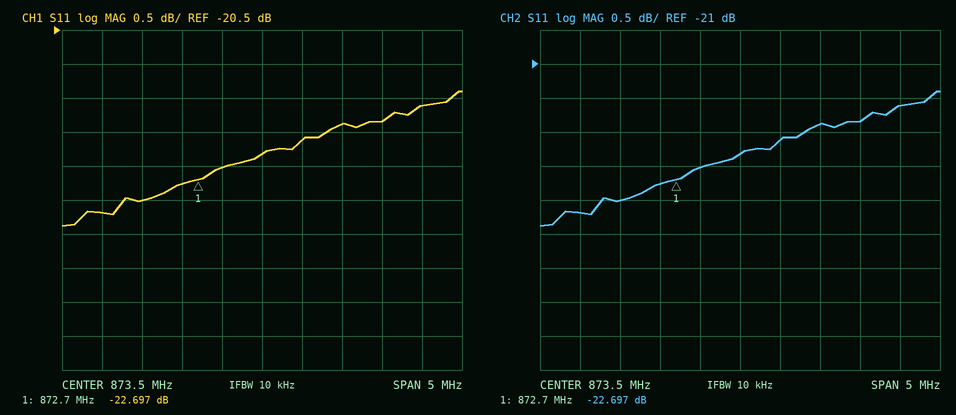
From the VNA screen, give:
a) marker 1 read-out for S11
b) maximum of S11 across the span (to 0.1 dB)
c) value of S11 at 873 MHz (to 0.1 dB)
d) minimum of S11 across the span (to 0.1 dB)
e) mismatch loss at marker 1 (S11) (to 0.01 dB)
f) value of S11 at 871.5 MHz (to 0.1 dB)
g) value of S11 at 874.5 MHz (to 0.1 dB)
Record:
-22.697 dB
-21.4 dB
-22.5 dB
-23.4 dB
0.02 dB
-23.2 dB
-21.9 dB
